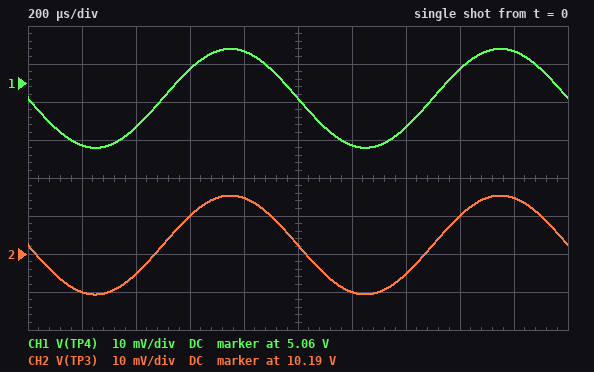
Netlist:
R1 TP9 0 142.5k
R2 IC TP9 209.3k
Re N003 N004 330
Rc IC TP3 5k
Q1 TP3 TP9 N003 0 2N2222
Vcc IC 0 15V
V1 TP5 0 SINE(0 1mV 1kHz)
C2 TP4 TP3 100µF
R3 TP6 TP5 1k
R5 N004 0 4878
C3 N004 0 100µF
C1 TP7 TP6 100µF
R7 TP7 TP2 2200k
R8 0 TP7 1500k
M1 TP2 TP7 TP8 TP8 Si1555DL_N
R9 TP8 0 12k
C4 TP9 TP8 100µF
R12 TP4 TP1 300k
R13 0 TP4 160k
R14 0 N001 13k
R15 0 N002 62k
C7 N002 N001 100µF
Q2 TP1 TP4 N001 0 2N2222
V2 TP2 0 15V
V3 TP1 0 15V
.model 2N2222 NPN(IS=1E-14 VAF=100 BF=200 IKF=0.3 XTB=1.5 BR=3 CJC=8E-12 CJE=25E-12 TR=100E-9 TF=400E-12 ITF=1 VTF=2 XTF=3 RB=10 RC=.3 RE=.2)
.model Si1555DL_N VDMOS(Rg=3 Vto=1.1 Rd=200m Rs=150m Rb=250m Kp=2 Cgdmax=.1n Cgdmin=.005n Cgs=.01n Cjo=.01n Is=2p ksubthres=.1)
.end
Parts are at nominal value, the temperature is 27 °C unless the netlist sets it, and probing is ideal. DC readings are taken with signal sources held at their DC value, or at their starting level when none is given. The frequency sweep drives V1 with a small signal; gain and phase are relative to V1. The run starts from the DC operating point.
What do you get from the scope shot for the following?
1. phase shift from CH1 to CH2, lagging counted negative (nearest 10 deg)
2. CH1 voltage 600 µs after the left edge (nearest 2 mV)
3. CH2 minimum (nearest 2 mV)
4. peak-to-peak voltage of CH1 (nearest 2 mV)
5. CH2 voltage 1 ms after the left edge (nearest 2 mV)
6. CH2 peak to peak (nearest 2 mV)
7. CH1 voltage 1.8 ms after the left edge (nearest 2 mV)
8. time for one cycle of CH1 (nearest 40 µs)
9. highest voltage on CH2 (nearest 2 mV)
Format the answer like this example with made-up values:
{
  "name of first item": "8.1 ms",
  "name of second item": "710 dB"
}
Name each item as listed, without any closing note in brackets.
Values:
{
  "phase shift from CH1 to CH2, lagging counted negative": "0 deg",
  "CH1 voltage 600 µs after the left edge": "5.064 V",
  "CH2 minimum": "10.180 V",
  "peak-to-peak voltage of CH1": "26 mV",
  "CH2 voltage 1 ms after the left edge": "10.192 V",
  "CH2 peak to peak": "26 mV",
  "CH1 voltage 1.8 ms after the left edge": "5.068 V",
  "time for one cycle of CH1": "1.00 ms",
  "highest voltage on CH2": "10.206 V"
}
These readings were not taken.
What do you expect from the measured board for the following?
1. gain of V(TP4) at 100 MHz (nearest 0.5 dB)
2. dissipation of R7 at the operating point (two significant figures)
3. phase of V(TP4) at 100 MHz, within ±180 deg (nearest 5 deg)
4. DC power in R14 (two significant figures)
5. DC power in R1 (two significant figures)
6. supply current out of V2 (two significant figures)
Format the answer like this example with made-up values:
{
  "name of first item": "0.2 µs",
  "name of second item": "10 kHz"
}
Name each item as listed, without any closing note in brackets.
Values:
{
  "gain of V(TP4) at 100 MHz": "-22.0 dB",
  "dissipation of R7 at the operating point": "36 µW",
  "phase of V(TP4) at 100 MHz, within ±180 deg": "-65 deg",
  "DC power in R14": "1.5 mW",
  "DC power in R1": "230 µW",
  "supply current out of V2": "430 µA"
}
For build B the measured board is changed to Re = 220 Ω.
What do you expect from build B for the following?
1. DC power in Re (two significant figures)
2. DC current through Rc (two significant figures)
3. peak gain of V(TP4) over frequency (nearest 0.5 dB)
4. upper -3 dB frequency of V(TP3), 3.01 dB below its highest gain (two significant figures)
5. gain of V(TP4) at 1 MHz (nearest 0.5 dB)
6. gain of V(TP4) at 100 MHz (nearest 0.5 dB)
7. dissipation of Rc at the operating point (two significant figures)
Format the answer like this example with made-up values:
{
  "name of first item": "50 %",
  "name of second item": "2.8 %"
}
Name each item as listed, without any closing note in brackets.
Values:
{
  "DC power in Re": "210 µW",
  "DC current through Rc": "980 µA",
  "peak gain of V(TP4) over frequency": "25.5 dB",
  "upper -3 dB frequency of V(TP3), 3.01 dB below its highest gain": "3.2 MHz",
  "gain of V(TP4) at 1 MHz": "25.0 dB",
  "gain of V(TP4) at 100 MHz": "-21.0 dB",
  "dissipation of Rc at the operating point": "4.8 mW"
}
